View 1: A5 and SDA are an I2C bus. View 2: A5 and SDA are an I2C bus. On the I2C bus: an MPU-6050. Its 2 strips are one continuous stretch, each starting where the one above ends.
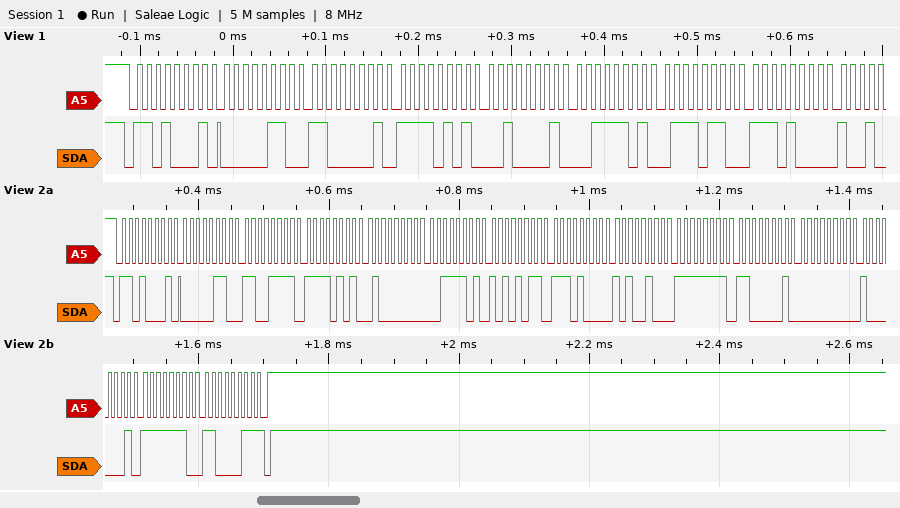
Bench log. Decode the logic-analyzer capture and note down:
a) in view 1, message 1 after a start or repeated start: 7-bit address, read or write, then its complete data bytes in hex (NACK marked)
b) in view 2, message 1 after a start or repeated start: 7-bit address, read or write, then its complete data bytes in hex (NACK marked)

0x68 read: 06 C1 F5 21 3D 76 E8
0x68 read: 06 CF F5 40 3D AB E8 A4 FF C1 00 81 FE C3 NACK
